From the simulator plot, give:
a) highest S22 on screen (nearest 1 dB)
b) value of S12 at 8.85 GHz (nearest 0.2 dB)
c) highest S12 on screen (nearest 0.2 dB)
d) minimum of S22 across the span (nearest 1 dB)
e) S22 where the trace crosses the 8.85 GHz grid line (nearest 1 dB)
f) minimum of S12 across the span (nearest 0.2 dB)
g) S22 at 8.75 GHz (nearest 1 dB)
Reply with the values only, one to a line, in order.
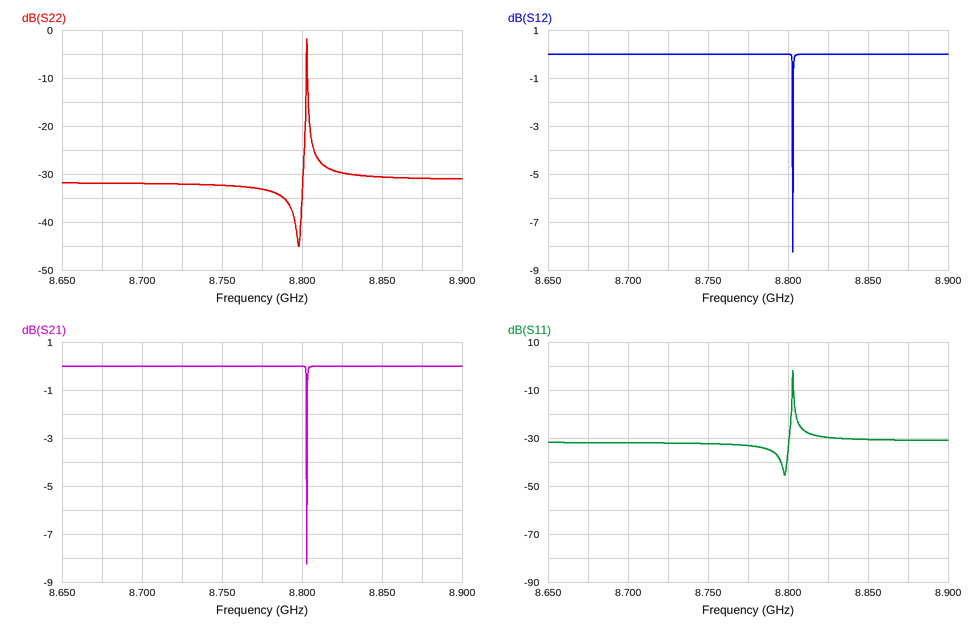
-2 dB
0.0 dB
0.0 dB
-45 dB
-31 dB
-8.2 dB
-32 dB
